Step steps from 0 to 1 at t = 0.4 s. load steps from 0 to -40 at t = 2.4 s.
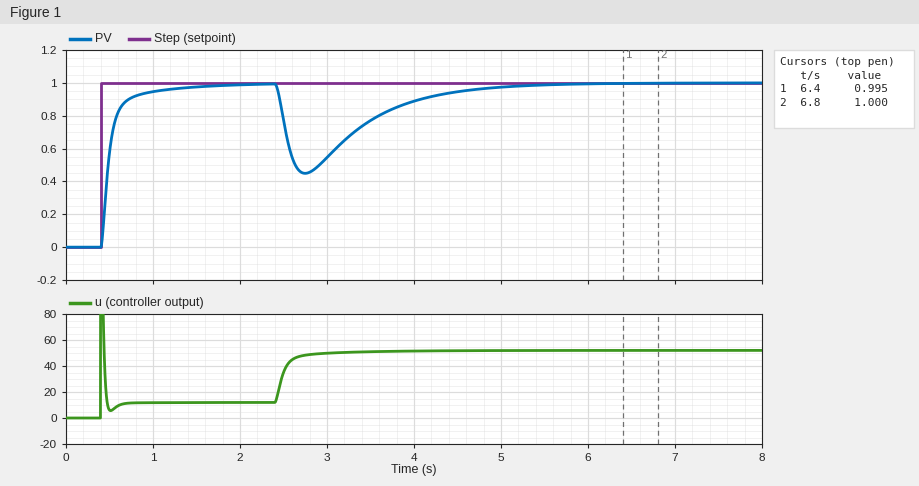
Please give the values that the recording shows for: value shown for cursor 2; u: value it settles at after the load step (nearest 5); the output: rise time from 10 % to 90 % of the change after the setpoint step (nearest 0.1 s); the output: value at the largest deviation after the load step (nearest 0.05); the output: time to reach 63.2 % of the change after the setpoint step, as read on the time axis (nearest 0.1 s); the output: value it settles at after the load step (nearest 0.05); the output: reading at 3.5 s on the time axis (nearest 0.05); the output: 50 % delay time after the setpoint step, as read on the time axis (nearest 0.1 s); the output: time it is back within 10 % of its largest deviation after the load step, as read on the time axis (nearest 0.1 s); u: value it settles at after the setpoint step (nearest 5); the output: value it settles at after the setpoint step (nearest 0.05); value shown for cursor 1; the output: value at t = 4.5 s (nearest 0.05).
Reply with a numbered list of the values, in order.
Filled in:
1. 1.000
2. 50
3. 0.3 s
4. 0.45
5. 0.5 s
6. 1.00
7. 0.75
8. 0.5 s
9. 4.5 s
10. 10
11. 1.00
12. 0.995
13. 0.95
